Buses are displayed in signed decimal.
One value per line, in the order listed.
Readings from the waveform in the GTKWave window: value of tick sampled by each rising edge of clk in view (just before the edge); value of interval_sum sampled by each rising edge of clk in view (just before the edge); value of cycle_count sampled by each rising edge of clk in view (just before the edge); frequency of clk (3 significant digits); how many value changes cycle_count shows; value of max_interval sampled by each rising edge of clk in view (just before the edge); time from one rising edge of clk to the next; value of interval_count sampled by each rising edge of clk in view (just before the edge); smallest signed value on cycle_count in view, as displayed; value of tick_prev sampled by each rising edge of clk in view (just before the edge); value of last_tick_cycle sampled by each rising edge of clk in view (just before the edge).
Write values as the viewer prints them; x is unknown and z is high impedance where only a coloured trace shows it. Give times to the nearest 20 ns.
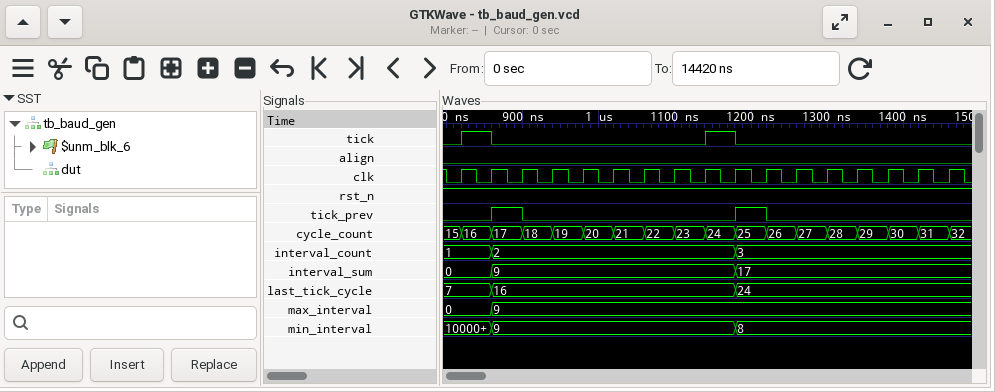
0 1 0 0 0 0 0 0 0 1 0 0 0 0 0 0 0
0, 0, 9, 9, 9, 9, 9, 9, 9, 9, 17, 17, 17, 17, 17, 17, 17
15, 16, 17, 18, 19, 20, 21, 22, 23, 24, 25, 26, 27, 28, 29, 30, 31
25.0 MHz
17
0, 0, 9, 9, 9, 9, 9, 9, 9, 9, 9, 9, 9, 9, 9, 9, 9
40 ns
1, 1, 2, 2, 2, 2, 2, 2, 2, 2, 3, 3, 3, 3, 3, 3, 3
15
0 0 1 0 0 0 0 0 0 0 1 0 0 0 0 0 0
7, 7, 16, 16, 16, 16, 16, 16, 16, 16, 24, 24, 24, 24, 24, 24, 24
